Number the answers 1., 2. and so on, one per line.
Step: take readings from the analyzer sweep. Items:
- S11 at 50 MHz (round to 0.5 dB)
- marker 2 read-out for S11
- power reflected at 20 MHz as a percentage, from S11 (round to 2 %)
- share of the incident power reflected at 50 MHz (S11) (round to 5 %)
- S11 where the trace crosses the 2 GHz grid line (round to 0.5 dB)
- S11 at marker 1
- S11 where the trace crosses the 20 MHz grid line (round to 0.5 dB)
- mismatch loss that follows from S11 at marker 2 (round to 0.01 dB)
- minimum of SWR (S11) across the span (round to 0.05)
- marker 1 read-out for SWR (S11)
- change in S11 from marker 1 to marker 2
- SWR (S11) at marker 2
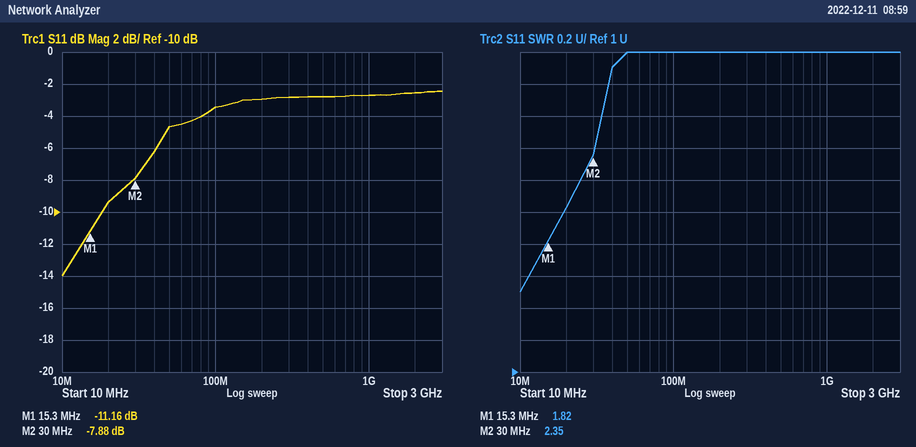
1. -4.5 dB
2. -7.88 dB
3. 12 %
4. 35 %
5. -2.5 dB
6. -11.16 dB
7. -9.5 dB
8. 0.77 dB
9. 1.50
10. 1.82
11. 3.28 dB
12. 2.35
